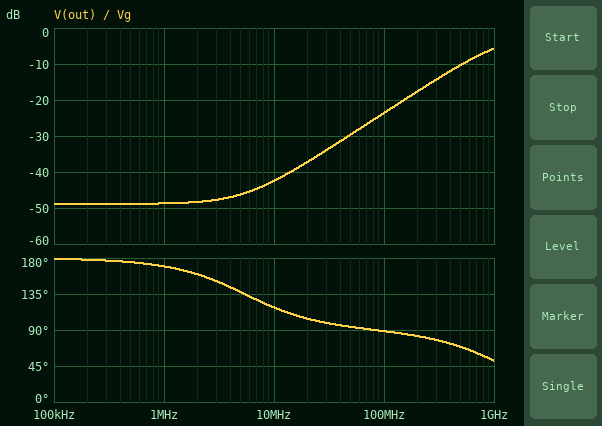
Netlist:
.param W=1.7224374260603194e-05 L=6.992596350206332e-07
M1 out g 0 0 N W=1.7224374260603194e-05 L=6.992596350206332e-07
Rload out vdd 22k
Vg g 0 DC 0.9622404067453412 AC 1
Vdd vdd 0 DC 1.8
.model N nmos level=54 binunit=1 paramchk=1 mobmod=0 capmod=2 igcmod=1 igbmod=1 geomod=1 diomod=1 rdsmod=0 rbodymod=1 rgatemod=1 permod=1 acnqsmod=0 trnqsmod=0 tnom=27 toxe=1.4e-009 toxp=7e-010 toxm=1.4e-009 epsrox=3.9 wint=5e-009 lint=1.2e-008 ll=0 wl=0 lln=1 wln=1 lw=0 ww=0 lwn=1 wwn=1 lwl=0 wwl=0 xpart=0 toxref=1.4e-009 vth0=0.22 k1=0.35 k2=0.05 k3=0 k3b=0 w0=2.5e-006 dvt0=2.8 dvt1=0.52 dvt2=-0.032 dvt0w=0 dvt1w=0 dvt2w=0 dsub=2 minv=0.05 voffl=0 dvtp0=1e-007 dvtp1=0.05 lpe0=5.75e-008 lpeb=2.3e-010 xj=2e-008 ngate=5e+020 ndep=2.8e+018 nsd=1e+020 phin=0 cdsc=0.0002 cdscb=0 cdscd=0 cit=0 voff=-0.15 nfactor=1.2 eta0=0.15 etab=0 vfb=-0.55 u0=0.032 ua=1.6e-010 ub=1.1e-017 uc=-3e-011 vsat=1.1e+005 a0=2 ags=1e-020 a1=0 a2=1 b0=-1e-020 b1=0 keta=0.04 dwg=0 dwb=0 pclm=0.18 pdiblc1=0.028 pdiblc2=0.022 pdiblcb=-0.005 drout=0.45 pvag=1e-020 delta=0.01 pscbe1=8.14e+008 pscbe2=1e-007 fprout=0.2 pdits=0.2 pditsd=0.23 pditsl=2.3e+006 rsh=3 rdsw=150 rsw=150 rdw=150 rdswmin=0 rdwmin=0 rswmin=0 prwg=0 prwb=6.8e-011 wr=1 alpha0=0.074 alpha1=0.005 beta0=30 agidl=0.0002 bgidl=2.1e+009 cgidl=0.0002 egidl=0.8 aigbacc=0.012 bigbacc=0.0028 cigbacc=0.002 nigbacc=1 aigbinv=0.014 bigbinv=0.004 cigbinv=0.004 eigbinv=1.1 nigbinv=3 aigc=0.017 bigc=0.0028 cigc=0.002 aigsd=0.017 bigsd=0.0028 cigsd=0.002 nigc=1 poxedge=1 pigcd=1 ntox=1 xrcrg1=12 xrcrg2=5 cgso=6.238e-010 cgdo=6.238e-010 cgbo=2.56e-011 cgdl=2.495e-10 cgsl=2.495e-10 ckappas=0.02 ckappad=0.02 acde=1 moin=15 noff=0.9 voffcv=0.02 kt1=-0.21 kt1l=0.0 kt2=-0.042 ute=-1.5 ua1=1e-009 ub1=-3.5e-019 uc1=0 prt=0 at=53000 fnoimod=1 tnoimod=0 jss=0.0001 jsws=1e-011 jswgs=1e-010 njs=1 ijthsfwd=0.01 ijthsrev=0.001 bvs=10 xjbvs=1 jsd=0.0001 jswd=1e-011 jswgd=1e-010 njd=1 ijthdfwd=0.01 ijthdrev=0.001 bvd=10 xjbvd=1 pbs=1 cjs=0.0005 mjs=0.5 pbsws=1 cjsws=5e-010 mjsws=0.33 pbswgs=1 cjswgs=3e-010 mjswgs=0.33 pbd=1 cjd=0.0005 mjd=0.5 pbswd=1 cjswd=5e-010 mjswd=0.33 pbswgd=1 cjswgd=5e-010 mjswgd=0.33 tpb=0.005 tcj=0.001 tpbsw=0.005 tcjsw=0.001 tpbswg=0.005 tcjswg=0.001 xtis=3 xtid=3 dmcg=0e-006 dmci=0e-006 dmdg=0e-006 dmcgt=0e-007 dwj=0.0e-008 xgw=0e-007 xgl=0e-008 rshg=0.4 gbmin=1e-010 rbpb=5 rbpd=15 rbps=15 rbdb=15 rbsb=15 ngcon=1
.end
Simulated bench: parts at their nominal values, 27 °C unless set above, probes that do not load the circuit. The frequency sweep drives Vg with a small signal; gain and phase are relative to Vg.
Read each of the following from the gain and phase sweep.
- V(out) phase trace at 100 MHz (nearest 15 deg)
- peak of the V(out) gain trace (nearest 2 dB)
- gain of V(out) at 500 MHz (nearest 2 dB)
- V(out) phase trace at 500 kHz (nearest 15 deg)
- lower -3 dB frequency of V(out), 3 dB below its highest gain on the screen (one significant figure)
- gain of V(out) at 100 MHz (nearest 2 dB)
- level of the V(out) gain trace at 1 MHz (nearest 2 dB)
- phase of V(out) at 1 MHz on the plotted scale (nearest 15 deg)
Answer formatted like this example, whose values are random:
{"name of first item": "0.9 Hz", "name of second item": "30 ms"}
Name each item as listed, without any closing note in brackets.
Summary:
{"V(out) phase trace at 100 MHz": "90 deg", "peak of the V(out) gain trace": "-6 dB", "gain of V(out) at 500 MHz": "-10 dB", "V(out) phase trace at 500 kHz": "180 deg", "lower -3 dB frequency of V(out), 3 dB below its highest gain on the screen": "600 MHz", "gain of V(out) at 100 MHz": "-24 dB", "level of the V(out) gain trace at 1 MHz": "-48 dB", "phase of V(out) at 1 MHz on the plotted scale": "165 deg"}
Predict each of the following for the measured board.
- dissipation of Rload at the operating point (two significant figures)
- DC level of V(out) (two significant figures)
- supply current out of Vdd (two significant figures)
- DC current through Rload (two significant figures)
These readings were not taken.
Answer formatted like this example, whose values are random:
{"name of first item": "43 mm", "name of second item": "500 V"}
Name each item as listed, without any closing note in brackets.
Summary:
{"dissipation of Rload at the operating point": "140 µW", "DC level of V(out)": "34 mV", "supply current out of Vdd": "80 µA", "DC current through Rload": "80 µA"}
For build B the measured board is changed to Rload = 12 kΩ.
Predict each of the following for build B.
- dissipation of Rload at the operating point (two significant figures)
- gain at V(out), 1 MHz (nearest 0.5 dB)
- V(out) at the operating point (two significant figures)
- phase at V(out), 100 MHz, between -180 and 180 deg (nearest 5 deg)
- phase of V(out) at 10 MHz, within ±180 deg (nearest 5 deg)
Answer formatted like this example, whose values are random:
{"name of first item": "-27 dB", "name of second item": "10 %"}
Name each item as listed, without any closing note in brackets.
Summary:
{"dissipation of Rload at the operating point": "250 µW", "gain at V(out), 1 MHz": "-40.0 dB", "V(out) at the operating point": "63 mV", "phase at V(out), 100 MHz, between -180 and 180 deg": "95 deg", "phase of V(out) at 10 MHz, within ±180 deg": "145 deg"}
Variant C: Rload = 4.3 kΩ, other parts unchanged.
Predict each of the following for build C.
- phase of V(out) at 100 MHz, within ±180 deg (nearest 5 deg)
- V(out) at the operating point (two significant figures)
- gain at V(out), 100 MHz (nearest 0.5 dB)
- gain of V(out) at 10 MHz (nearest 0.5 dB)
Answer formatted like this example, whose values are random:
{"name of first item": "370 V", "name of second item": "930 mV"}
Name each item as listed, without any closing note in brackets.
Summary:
{"phase of V(out) at 100 MHz, within ±180 deg": "130 deg", "V(out) at the operating point": "190 mV", "gain at V(out), 100 MHz": "-19.5 dB", "gain of V(out) at 10 MHz": "-22.5 dB"}
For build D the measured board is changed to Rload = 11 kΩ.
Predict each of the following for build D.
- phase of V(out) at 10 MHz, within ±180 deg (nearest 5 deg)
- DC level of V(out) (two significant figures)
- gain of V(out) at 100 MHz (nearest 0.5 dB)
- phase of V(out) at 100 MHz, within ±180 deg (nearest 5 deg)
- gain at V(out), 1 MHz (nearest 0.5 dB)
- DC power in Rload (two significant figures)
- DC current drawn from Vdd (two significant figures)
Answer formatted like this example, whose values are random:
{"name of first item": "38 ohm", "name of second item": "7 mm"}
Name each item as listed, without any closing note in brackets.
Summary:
{"phase of V(out) at 10 MHz, within ±180 deg": "150 deg", "DC level of V(out)": "69 mV", "gain of V(out) at 100 MHz": "-23.0 dB", "phase of V(out) at 100 MHz, within ±180 deg": "95 deg", "gain at V(out), 1 MHz": "-38.5 dB", "DC power in Rload": "270 µW", "DC current drawn from Vdd": "160 µA"}
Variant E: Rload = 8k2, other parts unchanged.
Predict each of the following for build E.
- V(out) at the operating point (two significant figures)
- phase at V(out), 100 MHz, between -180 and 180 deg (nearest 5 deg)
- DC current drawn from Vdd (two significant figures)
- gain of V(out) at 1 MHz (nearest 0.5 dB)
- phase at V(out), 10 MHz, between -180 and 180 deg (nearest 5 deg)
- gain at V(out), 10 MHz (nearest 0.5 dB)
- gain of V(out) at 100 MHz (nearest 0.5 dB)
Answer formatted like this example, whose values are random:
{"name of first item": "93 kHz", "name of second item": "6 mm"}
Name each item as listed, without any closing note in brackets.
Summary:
{"V(out) at the operating point": "93 mV", "phase at V(out), 100 MHz, between -180 and 180 deg": "100 deg", "DC current drawn from Vdd": "210 µA", "gain of V(out) at 1 MHz": "-34.0 dB", "phase at V(out), 10 MHz, between -180 and 180 deg": "160 deg", "gain at V(out), 10 MHz": "-33.5 dB", "gain of V(out) at 100 MHz": "-22.5 dB"}
